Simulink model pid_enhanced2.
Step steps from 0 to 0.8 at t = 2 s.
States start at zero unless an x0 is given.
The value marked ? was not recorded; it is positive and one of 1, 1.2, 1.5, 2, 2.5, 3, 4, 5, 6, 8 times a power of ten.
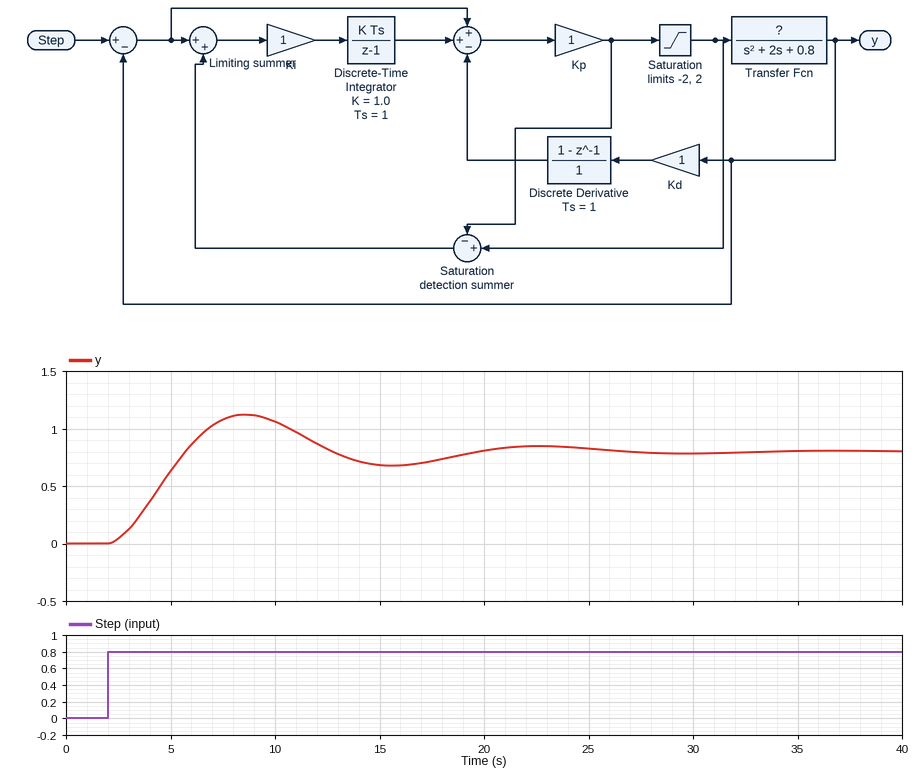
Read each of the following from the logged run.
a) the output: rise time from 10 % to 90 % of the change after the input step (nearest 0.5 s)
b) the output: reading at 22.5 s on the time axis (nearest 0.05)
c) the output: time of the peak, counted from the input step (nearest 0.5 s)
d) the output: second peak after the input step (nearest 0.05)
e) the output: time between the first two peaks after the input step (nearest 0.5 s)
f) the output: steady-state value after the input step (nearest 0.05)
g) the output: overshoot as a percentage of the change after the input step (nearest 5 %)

2.5 s
0.85
6.5 s
0.85
14.0 s
0.80
40 %
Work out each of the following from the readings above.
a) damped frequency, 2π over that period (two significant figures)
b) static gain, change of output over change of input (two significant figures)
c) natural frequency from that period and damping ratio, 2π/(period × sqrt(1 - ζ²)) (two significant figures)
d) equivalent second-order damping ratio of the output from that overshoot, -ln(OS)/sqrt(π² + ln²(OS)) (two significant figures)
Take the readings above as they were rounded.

0.45 rad/s
1.0
0.47 rad/s
0.28
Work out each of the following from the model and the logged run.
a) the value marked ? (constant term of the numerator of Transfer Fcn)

0.6
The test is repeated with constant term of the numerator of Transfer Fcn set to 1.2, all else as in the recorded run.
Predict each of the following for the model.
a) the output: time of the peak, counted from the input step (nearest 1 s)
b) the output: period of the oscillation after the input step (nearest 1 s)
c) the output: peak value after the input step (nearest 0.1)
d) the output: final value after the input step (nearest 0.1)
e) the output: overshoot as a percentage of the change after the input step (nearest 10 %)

5 s
11 s
1.2
0.8
50 %
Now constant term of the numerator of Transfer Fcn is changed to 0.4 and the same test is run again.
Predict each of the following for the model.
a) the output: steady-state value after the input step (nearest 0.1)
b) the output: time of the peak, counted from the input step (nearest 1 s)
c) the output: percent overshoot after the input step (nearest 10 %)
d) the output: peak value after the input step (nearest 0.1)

0.8
8 s
20 %
0.9
